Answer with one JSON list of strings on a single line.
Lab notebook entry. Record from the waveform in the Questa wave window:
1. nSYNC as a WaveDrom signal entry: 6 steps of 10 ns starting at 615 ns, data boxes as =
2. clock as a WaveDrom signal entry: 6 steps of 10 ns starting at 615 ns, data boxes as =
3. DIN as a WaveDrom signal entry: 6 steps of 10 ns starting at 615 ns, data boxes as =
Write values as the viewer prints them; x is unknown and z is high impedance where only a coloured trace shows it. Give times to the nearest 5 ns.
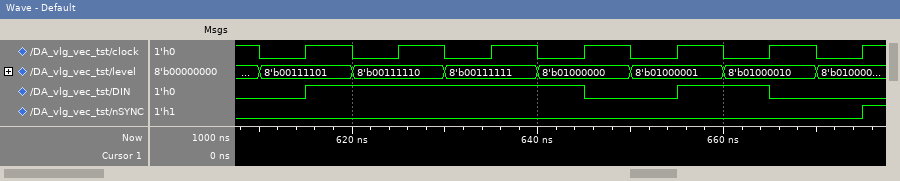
["{name: 'nSYNC', wave: '0.....'}", "{name: 'clock', wave: 'p.....'}", "{name: 'DIN', wave: '1..010'}"]
